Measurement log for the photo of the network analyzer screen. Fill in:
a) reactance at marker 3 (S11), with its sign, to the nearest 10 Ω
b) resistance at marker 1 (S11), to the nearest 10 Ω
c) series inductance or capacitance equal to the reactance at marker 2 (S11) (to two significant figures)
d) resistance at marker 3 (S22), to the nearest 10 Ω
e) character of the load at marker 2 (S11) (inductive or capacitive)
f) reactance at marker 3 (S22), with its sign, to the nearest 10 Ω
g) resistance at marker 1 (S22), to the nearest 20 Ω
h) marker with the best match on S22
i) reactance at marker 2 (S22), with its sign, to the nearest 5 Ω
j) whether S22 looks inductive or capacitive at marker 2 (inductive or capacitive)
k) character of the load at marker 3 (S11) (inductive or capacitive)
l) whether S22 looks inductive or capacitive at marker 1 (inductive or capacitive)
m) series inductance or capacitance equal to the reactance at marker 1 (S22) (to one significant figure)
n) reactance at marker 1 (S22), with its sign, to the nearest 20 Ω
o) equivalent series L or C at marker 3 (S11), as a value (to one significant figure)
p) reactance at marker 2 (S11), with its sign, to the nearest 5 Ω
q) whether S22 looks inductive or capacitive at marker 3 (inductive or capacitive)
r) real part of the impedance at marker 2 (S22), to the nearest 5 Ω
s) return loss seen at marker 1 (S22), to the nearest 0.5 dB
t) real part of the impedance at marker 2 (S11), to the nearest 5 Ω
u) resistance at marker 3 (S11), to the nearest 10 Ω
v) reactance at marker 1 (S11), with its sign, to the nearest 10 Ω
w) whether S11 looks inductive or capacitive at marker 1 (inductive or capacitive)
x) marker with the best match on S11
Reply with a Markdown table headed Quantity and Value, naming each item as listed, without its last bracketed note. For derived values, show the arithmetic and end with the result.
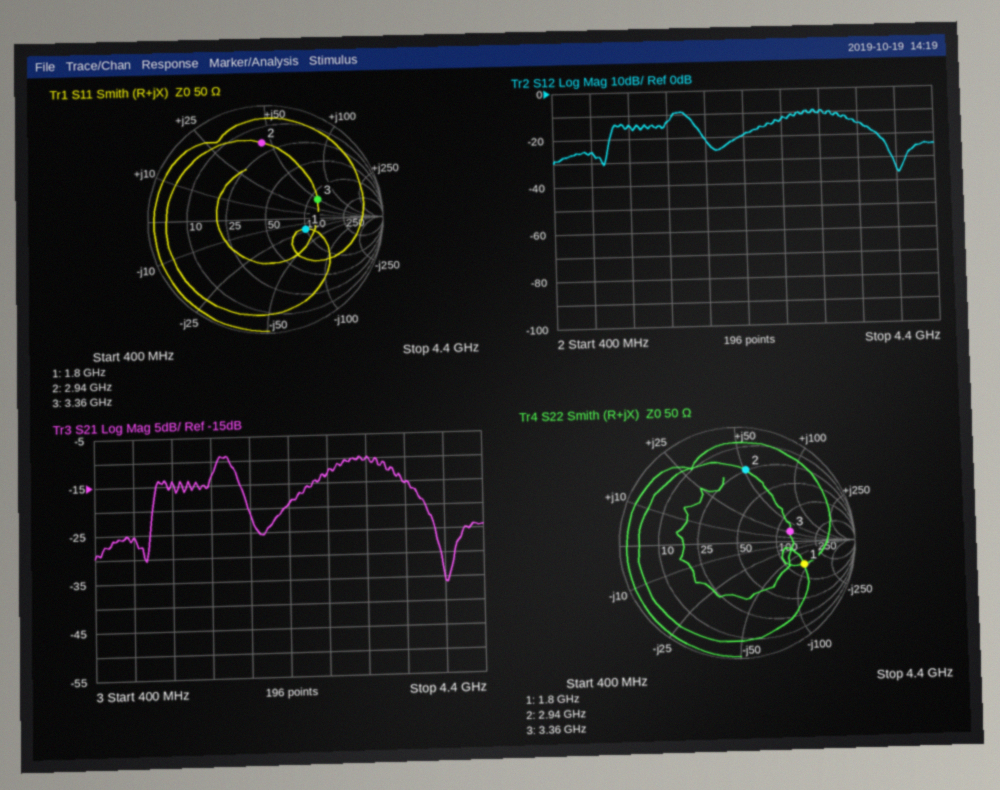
| Quantity | Value |
|---|---|
| reactance at marker 3 (S11), with its sign, to the nearest 10 Ω | +50 Ω |
| resistance at marker 1 (S11), to the nearest 10 Ω | 100 Ω |
| series inductance or capacitance equal to the reactance at marker 2 (S11) | L = 45 Ω/(2π × 2.94 GHz) ≈ 2.4 nH |
| resistance at marker 3 (S22), to the nearest 10 Ω | 130 Ω |
| character of the load at marker 2 (S11) | inductive |
| reactance at marker 3 (S22), with its sign, to the nearest 10 Ω | +30 Ω |
| resistance at marker 1 (S22), to the nearest 20 Ω | 140 Ω |
| marker with the best match on S22 | marker 3 |
| reactance at marker 2 (S22), with its sign, to the nearest 5 Ω | +50 Ω |
| whether S22 looks inductive or capacitive at marker 2 | inductive |
| character of the load at marker 3 (S11) | inductive |
| whether S22 looks inductive or capacitive at marker 1 | capacitive |
| series inductance or capacitance equal to the reactance at marker 1 (S22) | C = 1/(2π × 1.8 GHz × 80 Ω) ≈ 1 pF |
| reactance at marker 1 (S22), with its sign, to the nearest 20 Ω | -80 Ω |
| equivalent series L or C at marker 3 (S11), as a value | L = 50 Ω/(2π × 3.36 GHz) ≈ 2 nH |
| reactance at marker 2 (S11), with its sign, to the nearest 5 Ω | +45 Ω |
| whether S22 looks inductive or capacitive at marker 3 | inductive |
| real part of the impedance at marker 2 (S22), to the nearest 5 Ω | 25 Ω |
| return loss seen at marker 1 (S22), to the nearest 0.5 dB | 4.5 dB |
| real part of the impedance at marker 2 (S11), to the nearest 5 Ω | 20 Ω |
| resistance at marker 3 (S11), to the nearest 10 Ω | 120 Ω |
| reactance at marker 1 (S11), with its sign, to the nearest 10 Ω | -20 Ω |
| whether S11 looks inductive or capacitive at marker 1 | capacitive |
| marker with the best match on S11 | marker 1 |
